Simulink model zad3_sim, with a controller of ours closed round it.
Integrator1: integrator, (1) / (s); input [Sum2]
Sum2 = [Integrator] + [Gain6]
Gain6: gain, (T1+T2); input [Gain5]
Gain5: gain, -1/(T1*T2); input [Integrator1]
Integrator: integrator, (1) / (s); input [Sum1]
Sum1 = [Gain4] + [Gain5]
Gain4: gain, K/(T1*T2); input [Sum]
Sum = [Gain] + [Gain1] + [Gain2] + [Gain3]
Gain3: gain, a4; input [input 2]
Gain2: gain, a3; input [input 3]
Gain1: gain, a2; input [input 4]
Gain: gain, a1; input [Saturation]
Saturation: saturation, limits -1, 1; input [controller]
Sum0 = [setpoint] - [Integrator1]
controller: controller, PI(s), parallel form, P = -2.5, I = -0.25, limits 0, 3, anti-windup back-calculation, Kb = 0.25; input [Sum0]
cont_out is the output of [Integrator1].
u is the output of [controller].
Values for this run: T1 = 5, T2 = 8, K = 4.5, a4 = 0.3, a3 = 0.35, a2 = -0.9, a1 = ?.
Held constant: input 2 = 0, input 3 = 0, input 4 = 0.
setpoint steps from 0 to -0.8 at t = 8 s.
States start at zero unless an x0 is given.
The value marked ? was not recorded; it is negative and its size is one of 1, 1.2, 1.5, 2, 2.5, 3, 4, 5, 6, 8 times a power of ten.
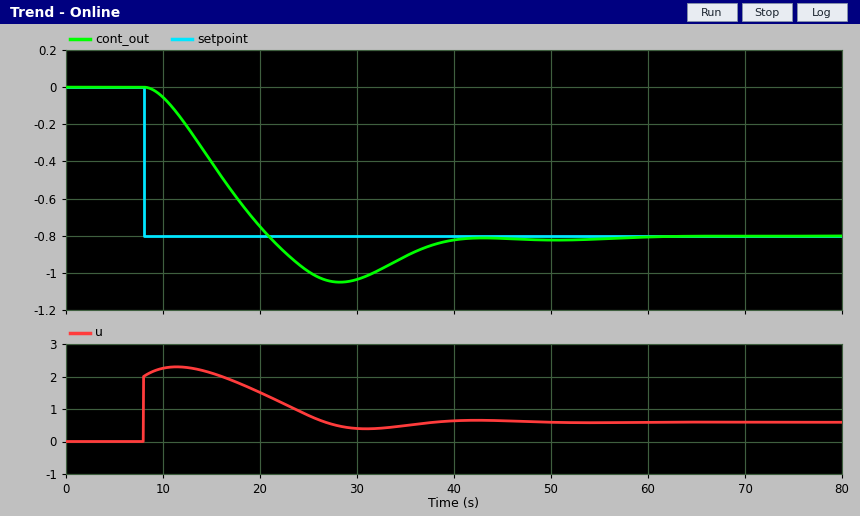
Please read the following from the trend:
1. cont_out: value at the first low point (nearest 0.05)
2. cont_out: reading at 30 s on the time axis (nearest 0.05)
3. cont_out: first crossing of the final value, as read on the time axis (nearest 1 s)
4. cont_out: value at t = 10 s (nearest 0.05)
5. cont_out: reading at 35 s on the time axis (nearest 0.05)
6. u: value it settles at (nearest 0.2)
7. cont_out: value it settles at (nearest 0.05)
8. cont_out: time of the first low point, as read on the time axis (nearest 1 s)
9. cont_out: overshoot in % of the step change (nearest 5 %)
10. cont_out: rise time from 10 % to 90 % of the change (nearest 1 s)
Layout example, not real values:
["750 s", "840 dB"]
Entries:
["-1.05", "-1.05", "21 s", "-0.05", "-0.90", "0.6", "-0.80", "28 s", "30 %", "9 s"]
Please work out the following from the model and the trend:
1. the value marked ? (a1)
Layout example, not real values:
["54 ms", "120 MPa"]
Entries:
["-0.3"]
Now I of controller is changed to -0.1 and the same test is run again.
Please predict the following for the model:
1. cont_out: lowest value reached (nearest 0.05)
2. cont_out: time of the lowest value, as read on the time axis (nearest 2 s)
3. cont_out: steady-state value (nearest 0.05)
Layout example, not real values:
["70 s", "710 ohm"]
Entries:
["-0.85", "24 s", "-0.80"]
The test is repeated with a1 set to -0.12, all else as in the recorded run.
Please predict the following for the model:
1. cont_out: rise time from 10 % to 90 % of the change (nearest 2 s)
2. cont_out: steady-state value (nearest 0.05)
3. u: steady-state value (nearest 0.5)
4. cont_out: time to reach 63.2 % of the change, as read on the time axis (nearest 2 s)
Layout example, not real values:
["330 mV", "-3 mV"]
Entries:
["22 s", "-0.55", "3.0", "22 s"]
